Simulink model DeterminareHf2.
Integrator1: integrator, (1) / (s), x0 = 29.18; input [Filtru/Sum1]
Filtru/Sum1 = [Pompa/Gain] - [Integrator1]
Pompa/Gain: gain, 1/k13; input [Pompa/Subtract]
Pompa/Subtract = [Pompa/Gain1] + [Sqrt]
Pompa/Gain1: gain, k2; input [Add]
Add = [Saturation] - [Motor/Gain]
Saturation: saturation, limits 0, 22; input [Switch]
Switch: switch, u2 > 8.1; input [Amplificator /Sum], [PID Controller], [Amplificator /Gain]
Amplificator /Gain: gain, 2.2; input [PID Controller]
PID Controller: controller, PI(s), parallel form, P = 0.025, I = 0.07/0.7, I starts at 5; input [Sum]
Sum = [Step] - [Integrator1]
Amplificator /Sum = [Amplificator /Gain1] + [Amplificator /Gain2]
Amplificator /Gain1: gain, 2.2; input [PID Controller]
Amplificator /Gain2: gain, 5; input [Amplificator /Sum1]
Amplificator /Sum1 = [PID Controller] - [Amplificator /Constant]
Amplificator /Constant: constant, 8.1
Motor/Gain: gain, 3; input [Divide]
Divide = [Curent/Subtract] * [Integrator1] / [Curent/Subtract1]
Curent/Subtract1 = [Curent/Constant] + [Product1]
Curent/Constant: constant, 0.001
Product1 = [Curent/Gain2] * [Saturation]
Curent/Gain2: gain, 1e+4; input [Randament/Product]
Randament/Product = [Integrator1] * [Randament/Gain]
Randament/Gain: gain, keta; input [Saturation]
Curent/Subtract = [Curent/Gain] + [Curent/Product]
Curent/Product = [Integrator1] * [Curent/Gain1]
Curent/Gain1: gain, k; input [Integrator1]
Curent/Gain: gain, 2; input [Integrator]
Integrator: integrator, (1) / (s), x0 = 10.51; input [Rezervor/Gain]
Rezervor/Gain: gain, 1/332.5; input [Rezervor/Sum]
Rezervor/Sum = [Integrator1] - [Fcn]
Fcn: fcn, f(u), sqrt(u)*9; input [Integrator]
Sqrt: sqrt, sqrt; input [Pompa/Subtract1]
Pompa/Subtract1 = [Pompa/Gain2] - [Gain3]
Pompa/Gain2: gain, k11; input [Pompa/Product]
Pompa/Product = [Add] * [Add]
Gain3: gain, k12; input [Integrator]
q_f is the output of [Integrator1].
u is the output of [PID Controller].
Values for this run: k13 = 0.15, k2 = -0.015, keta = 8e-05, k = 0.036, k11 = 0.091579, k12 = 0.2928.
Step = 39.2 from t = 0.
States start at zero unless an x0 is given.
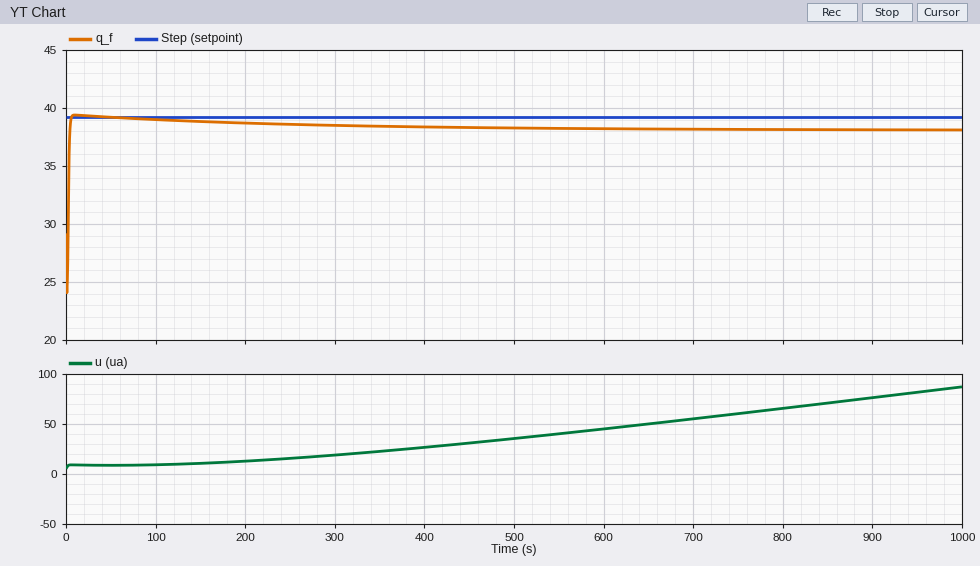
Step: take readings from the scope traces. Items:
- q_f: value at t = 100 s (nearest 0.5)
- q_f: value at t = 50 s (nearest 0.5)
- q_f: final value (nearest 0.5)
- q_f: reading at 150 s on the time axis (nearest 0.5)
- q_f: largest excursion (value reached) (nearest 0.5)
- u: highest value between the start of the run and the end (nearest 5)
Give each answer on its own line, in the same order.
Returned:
39.0
39.0
38.0
39.0
39.5
85
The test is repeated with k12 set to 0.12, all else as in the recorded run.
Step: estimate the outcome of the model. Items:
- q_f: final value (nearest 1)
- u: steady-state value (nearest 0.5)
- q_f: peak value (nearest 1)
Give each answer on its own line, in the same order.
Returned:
39
8.5
40
